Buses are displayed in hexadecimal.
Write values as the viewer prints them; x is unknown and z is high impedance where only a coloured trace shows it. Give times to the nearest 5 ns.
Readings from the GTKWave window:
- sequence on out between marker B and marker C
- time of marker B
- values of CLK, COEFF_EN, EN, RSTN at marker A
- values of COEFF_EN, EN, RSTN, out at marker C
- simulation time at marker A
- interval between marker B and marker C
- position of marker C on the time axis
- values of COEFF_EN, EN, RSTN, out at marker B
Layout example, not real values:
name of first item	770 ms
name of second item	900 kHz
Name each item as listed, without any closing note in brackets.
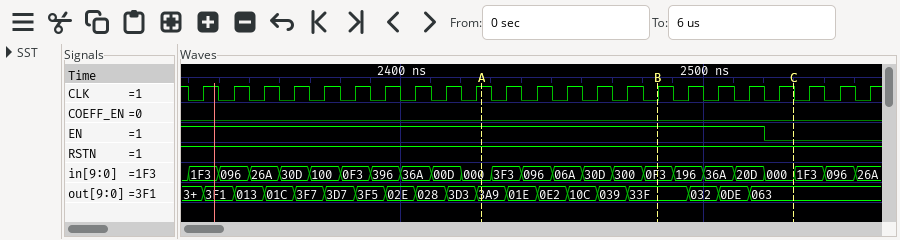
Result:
sequence on out between marker B and marker C	33F, 032, 0DE, 063
time of marker B	2485 ns
values of CLK, COEFF_EN, EN, RSTN at marker A	CLK=1, COEFF_EN=0, EN=1, RSTN=1
values of COEFF_EN, EN, RSTN, out at marker C	COEFF_EN=0, EN=0, RSTN=1, out=063
simulation time at marker A	2425 ns
interval between marker B and marker C	45 ns
position of marker C on the time axis	2530 ns
values of COEFF_EN, EN, RSTN, out at marker B	COEFF_EN=0, EN=1, RSTN=1, out=33F
